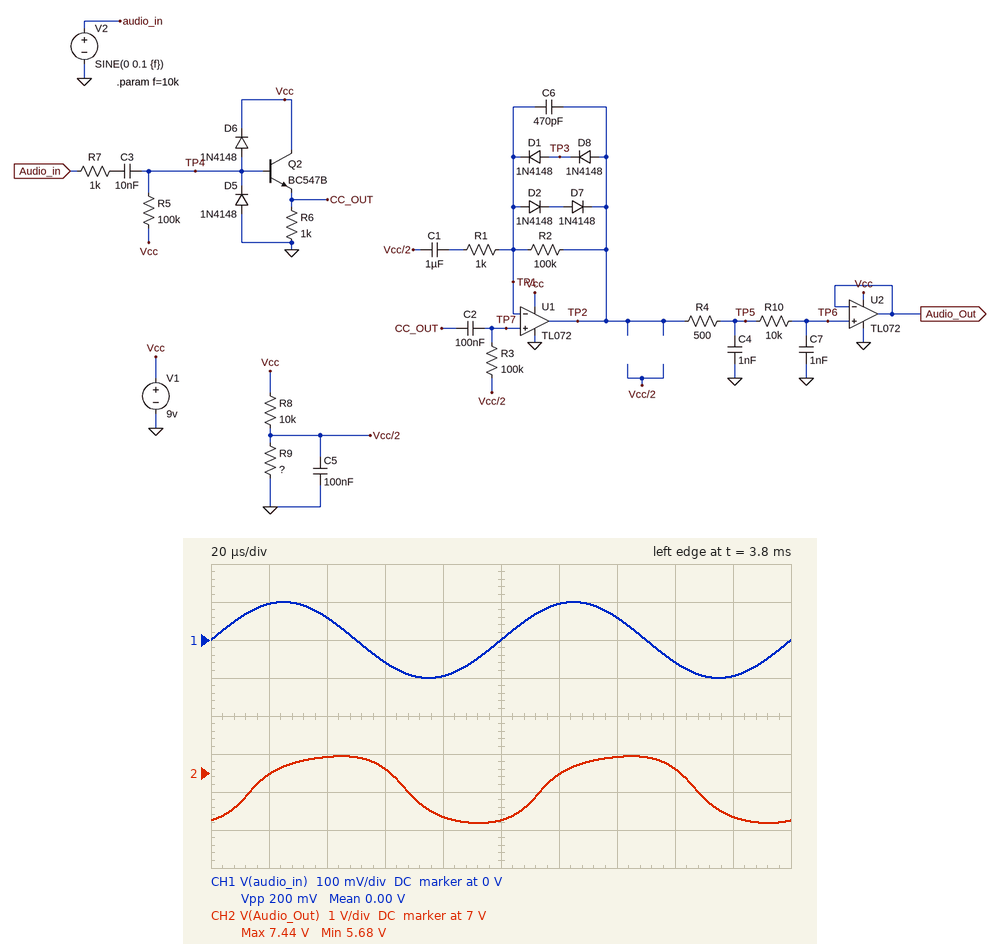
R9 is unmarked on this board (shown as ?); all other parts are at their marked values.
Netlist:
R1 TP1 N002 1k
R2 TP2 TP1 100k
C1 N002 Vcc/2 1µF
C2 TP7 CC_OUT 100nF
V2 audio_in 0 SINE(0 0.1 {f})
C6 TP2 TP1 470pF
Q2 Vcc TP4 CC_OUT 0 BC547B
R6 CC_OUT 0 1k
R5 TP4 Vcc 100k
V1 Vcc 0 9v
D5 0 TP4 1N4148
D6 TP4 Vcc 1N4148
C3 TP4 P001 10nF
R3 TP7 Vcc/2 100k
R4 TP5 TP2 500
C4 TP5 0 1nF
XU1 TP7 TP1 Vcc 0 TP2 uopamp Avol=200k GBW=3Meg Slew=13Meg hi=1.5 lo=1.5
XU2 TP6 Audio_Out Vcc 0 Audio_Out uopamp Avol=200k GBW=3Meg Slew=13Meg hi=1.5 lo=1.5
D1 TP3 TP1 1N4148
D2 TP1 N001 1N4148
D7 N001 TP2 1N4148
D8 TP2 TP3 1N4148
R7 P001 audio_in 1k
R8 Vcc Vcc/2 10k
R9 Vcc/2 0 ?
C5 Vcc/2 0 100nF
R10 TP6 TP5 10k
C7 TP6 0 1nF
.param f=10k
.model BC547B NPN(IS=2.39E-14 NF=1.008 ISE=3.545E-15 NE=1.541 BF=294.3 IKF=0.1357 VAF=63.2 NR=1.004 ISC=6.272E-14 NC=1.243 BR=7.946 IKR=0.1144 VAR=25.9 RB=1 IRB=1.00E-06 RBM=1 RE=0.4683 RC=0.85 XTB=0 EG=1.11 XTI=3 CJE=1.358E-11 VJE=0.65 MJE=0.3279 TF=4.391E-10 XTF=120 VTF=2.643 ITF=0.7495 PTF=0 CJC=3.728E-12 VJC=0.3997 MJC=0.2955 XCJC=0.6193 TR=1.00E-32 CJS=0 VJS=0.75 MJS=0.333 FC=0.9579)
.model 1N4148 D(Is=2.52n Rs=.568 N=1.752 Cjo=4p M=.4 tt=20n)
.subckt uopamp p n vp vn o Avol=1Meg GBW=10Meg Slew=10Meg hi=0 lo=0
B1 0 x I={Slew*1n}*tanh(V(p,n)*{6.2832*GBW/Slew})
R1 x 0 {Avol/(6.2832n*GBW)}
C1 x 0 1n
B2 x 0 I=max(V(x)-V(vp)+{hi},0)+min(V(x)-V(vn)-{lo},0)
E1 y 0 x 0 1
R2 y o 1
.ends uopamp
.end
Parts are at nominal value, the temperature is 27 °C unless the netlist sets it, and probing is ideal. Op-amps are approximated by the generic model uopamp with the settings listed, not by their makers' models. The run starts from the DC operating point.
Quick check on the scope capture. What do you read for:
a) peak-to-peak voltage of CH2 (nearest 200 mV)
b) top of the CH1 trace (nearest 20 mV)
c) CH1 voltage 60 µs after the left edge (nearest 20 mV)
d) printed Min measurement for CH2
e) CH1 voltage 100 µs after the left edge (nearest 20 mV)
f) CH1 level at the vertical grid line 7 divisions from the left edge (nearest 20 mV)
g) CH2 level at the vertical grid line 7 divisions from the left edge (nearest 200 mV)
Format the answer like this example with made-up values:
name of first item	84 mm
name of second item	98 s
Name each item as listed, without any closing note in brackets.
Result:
peak-to-peak voltage of CH2	1.8 V
top of the CH1 trace	100 mV
CH1 voltage 60 µs after the left edge	-60 mV
printed Min measurement for CH2	5.68 V
CH1 voltage 100 µs after the left edge	0 V
CH1 level at the vertical grid line 7 divisions from the left edge	60 mV
CH2 level at the vertical grid line 7 divisions from the left edge	7.4 V
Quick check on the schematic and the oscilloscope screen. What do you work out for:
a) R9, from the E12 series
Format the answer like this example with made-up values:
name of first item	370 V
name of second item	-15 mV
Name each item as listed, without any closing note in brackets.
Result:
R9, from the E12 series	27 kΩ
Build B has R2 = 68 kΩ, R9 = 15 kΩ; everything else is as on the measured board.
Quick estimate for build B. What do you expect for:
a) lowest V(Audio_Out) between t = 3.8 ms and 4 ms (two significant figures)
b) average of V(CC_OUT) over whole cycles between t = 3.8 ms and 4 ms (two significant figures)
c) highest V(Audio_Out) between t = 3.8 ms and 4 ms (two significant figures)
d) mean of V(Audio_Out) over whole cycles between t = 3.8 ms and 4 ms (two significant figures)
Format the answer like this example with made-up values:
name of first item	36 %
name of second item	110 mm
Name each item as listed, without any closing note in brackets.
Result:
lowest V(Audio_Out) between t = 3.8 ms and 4 ms	4.5 V
average of V(CC_OUT) over whole cycles between t = 3.8 ms and 4 ms	6.1 V
highest V(Audio_Out) between t = 3.8 ms and 4 ms	6.3 V
mean of V(Audio_Out) over whole cycles between t = 3.8 ms and 4 ms	5.4 V
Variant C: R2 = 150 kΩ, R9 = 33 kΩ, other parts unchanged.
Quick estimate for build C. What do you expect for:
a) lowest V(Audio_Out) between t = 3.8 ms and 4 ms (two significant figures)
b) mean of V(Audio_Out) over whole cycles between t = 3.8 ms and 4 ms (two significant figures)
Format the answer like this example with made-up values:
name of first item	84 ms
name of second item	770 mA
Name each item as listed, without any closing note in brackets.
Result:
lowest V(Audio_Out) between t = 3.8 ms and 4 ms	6.1 V
mean of V(Audio_Out) over whole cycles between t = 3.8 ms and 4 ms	7.0 V
